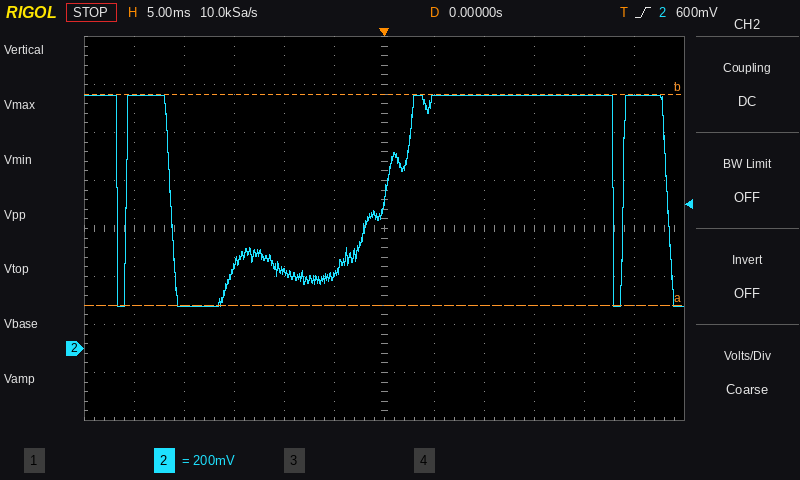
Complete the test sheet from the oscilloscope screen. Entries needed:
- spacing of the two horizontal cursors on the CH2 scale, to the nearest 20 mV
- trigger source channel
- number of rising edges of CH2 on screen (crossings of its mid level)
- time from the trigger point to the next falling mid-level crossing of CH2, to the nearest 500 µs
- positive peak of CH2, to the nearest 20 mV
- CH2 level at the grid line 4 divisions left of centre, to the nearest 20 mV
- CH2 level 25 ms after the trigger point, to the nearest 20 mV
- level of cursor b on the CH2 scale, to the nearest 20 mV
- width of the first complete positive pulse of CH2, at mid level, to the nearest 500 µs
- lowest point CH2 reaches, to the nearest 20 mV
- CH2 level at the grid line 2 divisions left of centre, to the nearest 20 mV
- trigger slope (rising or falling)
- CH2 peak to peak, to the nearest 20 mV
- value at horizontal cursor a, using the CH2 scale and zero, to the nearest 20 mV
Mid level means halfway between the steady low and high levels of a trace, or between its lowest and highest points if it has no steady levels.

880 mV
CH2
3
23.0 ms
1.06 V
180 mV
1.06 V
1.06 V
4.5 ms
180 mV
320 mV
rising
880 mV
180 mV
